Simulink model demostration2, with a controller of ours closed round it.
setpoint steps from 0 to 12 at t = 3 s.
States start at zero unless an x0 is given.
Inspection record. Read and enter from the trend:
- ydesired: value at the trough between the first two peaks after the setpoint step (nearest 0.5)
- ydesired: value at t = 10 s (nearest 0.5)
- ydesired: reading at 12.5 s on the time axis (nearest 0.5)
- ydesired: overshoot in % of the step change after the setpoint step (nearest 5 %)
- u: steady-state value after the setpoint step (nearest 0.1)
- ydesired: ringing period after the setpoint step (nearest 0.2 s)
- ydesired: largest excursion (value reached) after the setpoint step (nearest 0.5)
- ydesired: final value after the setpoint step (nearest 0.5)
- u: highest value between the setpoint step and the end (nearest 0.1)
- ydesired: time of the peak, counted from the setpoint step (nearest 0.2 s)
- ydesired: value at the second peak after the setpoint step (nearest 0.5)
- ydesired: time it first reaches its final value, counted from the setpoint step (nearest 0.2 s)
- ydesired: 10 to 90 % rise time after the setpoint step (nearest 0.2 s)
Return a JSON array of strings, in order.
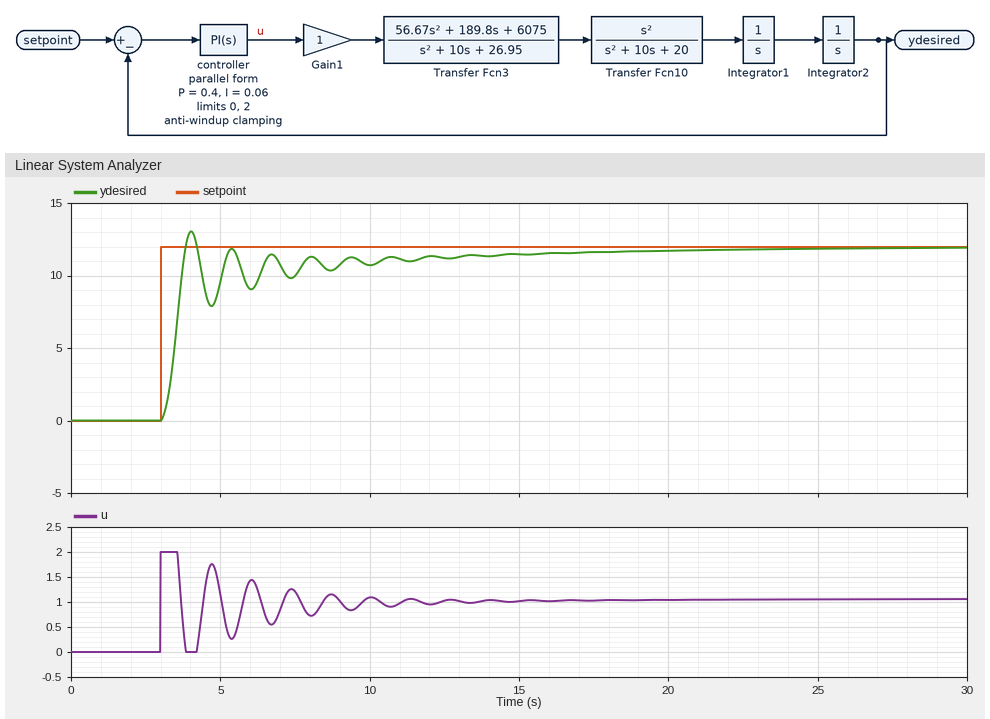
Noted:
["8.0", "10.5", "11.0", "10 %", "1.1", "1.4 s", "13.0", "12.0", "2.0", "1.0 s", "12.0", "0.8 s", "0.6 s"]
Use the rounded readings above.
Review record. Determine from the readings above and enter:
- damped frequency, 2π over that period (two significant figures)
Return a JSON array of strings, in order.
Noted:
["4.5 rad/s"]
